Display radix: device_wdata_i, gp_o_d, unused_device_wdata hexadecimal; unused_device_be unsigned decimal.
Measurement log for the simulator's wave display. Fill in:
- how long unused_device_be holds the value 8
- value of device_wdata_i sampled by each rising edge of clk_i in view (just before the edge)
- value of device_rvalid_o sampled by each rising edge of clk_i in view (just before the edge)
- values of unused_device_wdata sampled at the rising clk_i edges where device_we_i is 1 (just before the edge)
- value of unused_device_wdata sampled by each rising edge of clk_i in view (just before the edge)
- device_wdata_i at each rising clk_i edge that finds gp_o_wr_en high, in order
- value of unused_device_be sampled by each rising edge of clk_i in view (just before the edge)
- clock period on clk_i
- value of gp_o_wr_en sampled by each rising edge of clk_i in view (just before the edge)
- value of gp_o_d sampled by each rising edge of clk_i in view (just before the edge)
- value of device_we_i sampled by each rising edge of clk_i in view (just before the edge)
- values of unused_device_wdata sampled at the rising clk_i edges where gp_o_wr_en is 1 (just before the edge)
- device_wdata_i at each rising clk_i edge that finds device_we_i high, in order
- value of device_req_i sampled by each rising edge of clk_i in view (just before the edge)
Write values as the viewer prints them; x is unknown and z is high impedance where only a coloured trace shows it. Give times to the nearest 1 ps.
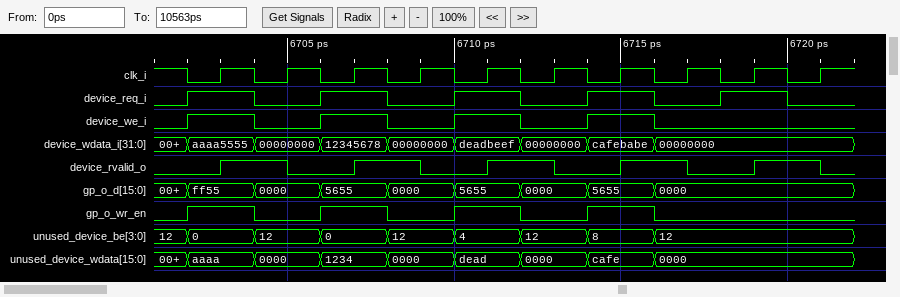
2 ps
aaaa5555, 00000000, 12345678, 00000000, deadbeef, 00000000, cafebabe, 00000000, 00000000, 00000000
0 1 0 1 0 1 0 1 0 1
aaaa, 1234, dead, cafe
aaaa, 0000, 1234, 0000, dead, 0000, cafe, 0000, 0000, 0000
aaaa5555, 12345678, deadbeef, cafebabe
0, 12, 0, 12, 4, 12, 8, 12, 12, 12
2 ps
1 0 1 0 1 0 1 0 0 0
ff55, 0000, 5655, 0000, 5655, 0000, 5655, 0000, 0000, 0000
1 0 1 0 1 0 1 0 0 0
aaaa, 1234, dead, cafe
aaaa5555, 12345678, deadbeef, cafebabe
1 0 1 0 1 0 1 0 1 0
